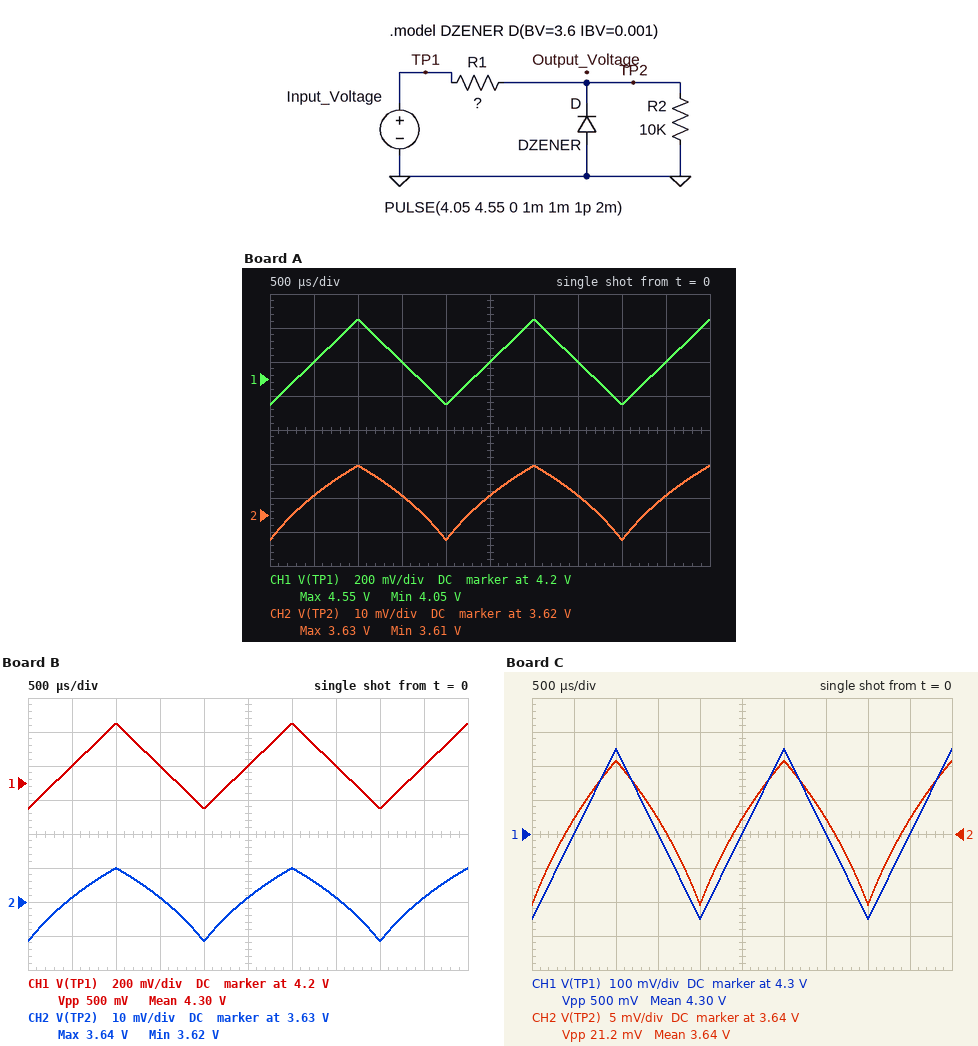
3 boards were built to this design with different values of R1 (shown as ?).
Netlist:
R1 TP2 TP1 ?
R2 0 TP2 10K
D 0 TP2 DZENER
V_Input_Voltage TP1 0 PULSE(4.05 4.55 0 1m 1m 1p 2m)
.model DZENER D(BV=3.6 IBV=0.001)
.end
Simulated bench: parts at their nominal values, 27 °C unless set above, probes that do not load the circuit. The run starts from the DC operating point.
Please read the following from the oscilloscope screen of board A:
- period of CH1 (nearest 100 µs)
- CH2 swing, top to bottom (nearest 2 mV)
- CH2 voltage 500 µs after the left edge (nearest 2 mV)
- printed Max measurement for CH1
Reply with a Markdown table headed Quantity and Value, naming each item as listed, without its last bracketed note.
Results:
| Quantity | Value |
|---|---|
| period of CH1 | 2.0 ms |
| CH2 swing, top to bottom | 22 mV |
| CH2 voltage 500 µs after the left edge | 3.626 V |
| printed Max measurement for CH1 | 4.55 V |
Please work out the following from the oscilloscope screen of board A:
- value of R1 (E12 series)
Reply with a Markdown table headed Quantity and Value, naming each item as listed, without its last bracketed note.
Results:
| Quantity | Value |
|---|---|
| value of R1 | 220 Ω |
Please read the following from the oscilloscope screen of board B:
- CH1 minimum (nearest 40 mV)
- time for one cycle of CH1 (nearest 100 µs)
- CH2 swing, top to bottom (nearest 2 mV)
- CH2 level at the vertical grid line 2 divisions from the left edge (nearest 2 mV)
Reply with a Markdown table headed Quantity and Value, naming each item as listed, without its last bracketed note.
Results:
| Quantity | Value |
|---|---|
| CH1 minimum | 4.04 V |
| time for one cycle of CH1 | 2.0 ms |
| CH2 swing, top to bottom | 22 mV |
| CH2 level at the vertical grid line 2 divisions from the left edge | 3.640 V |
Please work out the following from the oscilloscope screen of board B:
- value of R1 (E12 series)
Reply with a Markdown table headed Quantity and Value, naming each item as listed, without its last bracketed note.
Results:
| Quantity | Value |
|---|---|
| value of R1 | 180 Ω |
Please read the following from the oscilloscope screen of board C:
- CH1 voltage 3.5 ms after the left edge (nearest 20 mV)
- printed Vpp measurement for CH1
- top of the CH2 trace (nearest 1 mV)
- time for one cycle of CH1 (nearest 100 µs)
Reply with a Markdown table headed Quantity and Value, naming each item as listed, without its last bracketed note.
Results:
| Quantity | Value |
|---|---|
| CH1 voltage 3.5 ms after the left edge | 4.30 V |
| printed Vpp measurement for CH1 | 500 mV |
| top of the CH2 trace | 3.651 V |
| time for one cycle of CH1 | 2.0 ms |
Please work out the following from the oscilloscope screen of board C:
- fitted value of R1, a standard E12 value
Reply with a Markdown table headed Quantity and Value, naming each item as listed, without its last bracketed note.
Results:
| Quantity | Value |
|---|---|
| fitted value of R1, a standard E12 value | 120 Ω |
